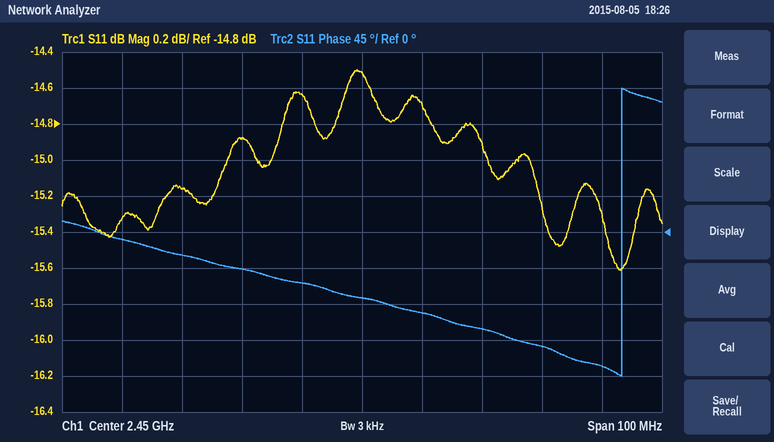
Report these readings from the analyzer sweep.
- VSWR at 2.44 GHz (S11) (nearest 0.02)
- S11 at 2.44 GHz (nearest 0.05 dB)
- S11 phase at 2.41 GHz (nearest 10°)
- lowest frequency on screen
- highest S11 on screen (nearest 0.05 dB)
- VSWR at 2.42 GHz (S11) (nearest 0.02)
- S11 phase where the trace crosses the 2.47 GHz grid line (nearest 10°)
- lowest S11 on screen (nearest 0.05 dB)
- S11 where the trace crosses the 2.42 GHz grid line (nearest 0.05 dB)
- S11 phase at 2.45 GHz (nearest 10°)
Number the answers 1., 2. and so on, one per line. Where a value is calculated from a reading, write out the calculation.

1. |Γ| = 10^(-14.65/20) = 0.1851; VSWR = (1 + 0.1851)/(1 − 0.1851) ≈ 1.45, so 1.46 to the nearest 0.02
2. -14.65 dB
3. -10°
4. 2.4 GHz
5. -14.50 dB
6. |Γ| = 10^(-15.15/20) = 0.1748; VSWR = (1 + 0.1748)/(1 − 0.1748) ≈ 1.42
7. -120°
8. -15.60 dB
9. -15.15 dB
10. -80°
